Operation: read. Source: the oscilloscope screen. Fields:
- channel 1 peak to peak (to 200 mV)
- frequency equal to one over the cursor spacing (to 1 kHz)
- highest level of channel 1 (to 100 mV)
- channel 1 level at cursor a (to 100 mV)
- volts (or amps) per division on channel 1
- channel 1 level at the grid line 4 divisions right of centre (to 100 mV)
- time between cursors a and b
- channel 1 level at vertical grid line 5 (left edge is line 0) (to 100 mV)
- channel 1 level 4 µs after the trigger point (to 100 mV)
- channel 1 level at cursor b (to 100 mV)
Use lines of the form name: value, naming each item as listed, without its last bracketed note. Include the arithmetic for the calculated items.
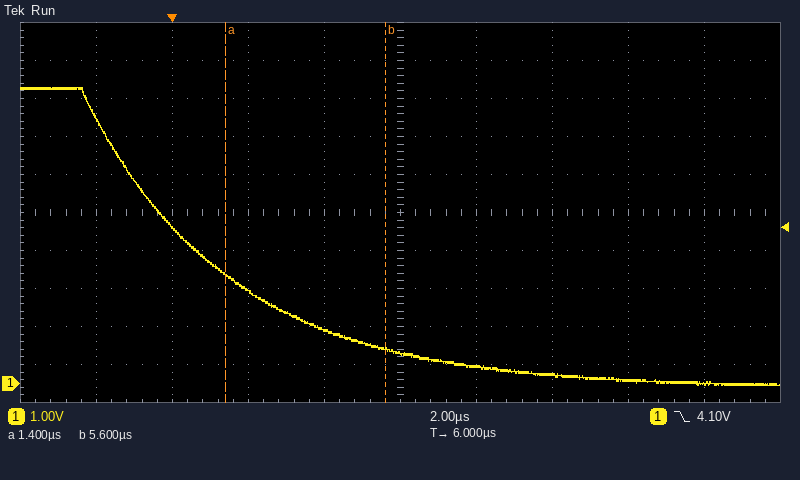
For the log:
channel 1 peak to peak: 7.8 V
frequency equal to one over the cursor spacing: 1 / 4.2 µs ≈ 238 kHz
highest level of channel 1: 7.8 V
channel 1 level at cursor a: 2.8 V
volts (or amps) per division on channel 1: 1 V
channel 1 level at the grid line 4 divisions right of centre: 0.0 V
time between cursors a and b: 5.6 µs − (1.4 µs) = 4.2 µs
channel 1 level at vertical grid line 5 (left edge is line 0): 800 mV
channel 1 level 4 µs after the trigger point: 1.4 V
channel 1 level at cursor b: 900 mV
